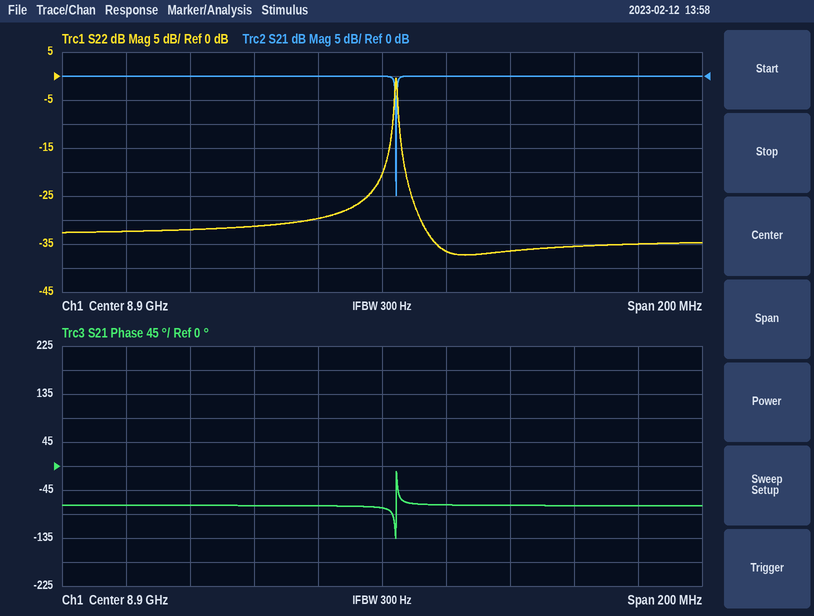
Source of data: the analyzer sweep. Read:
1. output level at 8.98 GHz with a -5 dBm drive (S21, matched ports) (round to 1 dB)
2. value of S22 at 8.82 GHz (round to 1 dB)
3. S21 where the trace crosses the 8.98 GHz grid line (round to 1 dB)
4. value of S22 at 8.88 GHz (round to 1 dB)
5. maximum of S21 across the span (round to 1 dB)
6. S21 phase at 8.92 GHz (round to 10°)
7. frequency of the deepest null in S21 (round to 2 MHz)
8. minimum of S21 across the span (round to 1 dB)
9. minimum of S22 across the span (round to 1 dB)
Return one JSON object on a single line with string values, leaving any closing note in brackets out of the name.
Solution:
{"output level at 8.98 GHz with a -5 dBm drive (S21, matched ports)": "-5 dBm", "value of S22 at 8.82 GHz": "-32 dB", "S21 where the trace crosses the 8.98 GHz grid line": "0 dB", "value of S22 at 8.88 GHz": "-30 dB", "maximum of S21 across the span": "0 dB", "S21 phase at 8.92 GHz": "-70°", "frequency of the deepest null in S21": "8.904 GHz", "minimum of S21 across the span": "-25 dB", "minimum of S22 across the span": "-37 dB"}
